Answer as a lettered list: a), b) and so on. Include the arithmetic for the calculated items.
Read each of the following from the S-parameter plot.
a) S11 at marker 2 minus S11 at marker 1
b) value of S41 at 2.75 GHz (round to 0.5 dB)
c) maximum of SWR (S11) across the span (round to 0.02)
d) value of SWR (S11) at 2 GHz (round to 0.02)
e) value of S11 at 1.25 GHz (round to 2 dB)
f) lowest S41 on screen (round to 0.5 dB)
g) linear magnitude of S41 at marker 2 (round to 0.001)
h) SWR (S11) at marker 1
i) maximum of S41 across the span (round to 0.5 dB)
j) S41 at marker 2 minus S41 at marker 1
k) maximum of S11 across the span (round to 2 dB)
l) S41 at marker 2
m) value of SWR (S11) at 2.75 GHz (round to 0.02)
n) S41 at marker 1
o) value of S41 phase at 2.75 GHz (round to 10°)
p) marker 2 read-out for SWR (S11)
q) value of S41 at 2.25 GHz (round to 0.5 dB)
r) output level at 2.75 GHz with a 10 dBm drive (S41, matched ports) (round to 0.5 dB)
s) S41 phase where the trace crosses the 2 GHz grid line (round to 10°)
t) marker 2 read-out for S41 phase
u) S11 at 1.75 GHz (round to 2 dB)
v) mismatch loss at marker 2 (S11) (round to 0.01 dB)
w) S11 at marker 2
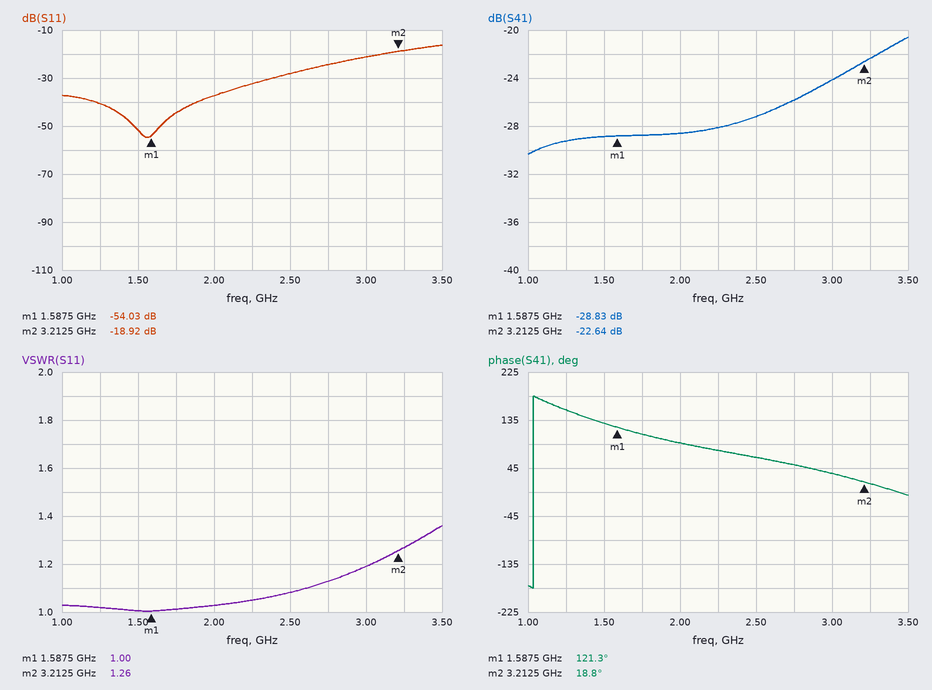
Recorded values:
a) -18.92 − (-54.03) = 35.11 dB
b) -26.0 dB
c) 1.36
d) 1.02
e) -40 dB
f) -30.5 dB
g) 10^(-22.64/20) ≈ 0.074
h) 1.00
i) -20.5 dB
j) -22.64 − (-28.83) = 6.19 dB
k) -16 dB
l) -22.64 dB
m) 1.12
n) -28.83 dB
o) 50°
p) 1.26
q) -28.0 dB
r) 10 dBm + (-26.0 dB) = -16.0 dBm
s) 90°
t) 18.8°
u) -44 dB
v) −10 log10(1 − 10^(-18.92/10)) ≈ 0.06 dB
w) -18.92 dB
